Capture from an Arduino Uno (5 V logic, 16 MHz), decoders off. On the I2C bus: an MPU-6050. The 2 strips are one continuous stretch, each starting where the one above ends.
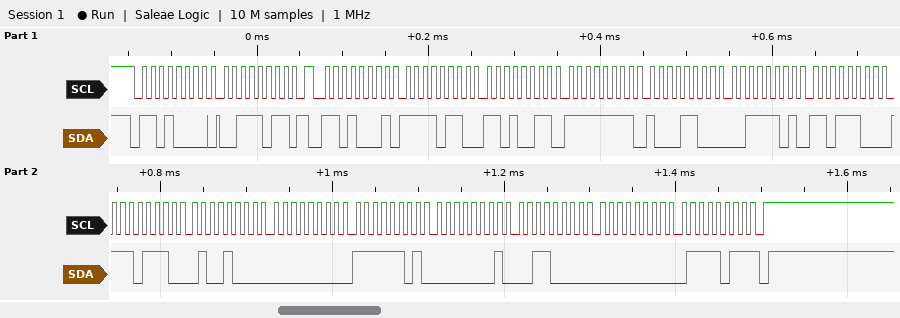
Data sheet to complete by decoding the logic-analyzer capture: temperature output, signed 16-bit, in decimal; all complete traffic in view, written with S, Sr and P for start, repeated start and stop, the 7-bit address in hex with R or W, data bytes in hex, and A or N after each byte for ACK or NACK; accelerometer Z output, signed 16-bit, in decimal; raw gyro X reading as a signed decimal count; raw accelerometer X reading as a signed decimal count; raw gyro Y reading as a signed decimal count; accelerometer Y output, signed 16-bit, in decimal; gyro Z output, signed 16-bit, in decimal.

-4536
S 68W A 3B A Sr 68R A F6 A D3 A FF A 8C A 3D A DC A EE A 48 A 00 A FD A 01 A 30 A 00 A 7B N P
15836
253
-2349
304
-116
123
